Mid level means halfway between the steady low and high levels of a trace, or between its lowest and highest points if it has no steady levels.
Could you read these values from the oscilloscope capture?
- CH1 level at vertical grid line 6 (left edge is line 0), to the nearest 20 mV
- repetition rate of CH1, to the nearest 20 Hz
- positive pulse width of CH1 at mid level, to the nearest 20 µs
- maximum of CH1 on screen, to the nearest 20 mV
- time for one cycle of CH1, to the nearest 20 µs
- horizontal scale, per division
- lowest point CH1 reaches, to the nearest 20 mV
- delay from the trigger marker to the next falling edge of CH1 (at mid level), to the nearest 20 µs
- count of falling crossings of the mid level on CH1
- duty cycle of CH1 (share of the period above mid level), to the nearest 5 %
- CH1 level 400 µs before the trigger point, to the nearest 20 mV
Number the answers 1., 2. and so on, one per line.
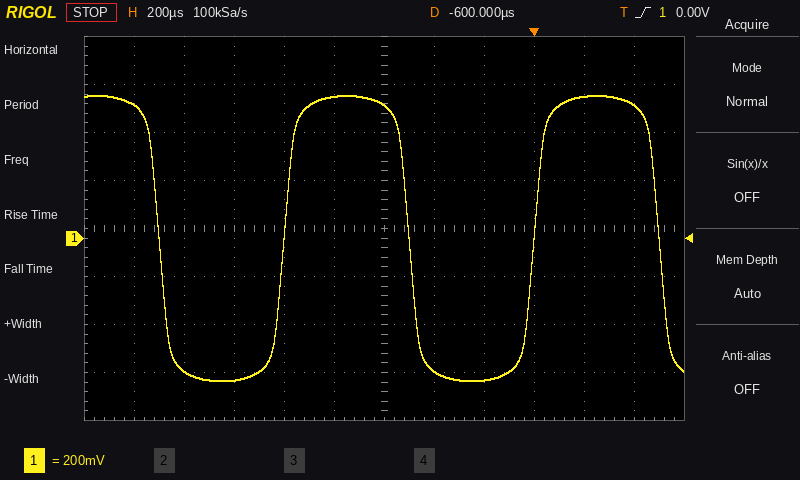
1. 560 mV
2. 1.00 kHz
3. 500 µs
4. 600 mV
5. 1.00 ms
6. 200 µs
7. -600 mV
8. 500 µs
9. 3
10. 50 %
11. -560 mV
